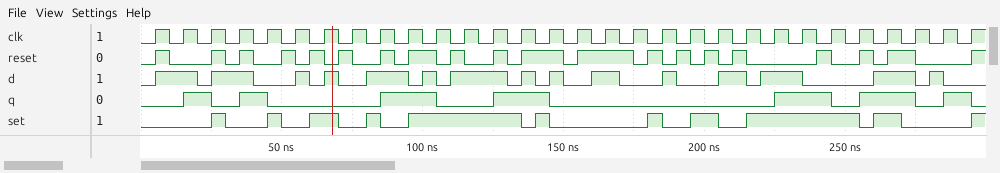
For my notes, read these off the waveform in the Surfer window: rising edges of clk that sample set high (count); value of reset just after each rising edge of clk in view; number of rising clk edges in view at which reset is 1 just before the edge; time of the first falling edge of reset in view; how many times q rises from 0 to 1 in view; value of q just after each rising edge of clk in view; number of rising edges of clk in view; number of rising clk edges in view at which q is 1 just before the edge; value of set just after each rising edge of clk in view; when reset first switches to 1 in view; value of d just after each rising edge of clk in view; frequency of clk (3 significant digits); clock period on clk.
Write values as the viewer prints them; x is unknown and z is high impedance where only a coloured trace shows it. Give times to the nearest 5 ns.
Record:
14
1 0 1 1 0 0 0 0 1 1 0 0 1 1 1 1 1 0 0 0 0 0 0 0 0 1 1 0 0 1
14
10 ns
7
0 1 0 1 0 0 0 0 1 1 0 0 1 1 0 0 0 0 0 0 0 0 1 1 0 1 1 0 1 0
30
11
0 0 1 0 1 0 1 0 0 1 1 1 1 0 0 0 0 0 0 1 0 1 1 1 1 0 1 0 0 1
5 ns
1 1 1 1 0 1 1 0 1 0 0 1 1 1 1 0 1 0 1 0 1 0 1 0 0 0 1 0 0 0
100 MHz
10 ns
